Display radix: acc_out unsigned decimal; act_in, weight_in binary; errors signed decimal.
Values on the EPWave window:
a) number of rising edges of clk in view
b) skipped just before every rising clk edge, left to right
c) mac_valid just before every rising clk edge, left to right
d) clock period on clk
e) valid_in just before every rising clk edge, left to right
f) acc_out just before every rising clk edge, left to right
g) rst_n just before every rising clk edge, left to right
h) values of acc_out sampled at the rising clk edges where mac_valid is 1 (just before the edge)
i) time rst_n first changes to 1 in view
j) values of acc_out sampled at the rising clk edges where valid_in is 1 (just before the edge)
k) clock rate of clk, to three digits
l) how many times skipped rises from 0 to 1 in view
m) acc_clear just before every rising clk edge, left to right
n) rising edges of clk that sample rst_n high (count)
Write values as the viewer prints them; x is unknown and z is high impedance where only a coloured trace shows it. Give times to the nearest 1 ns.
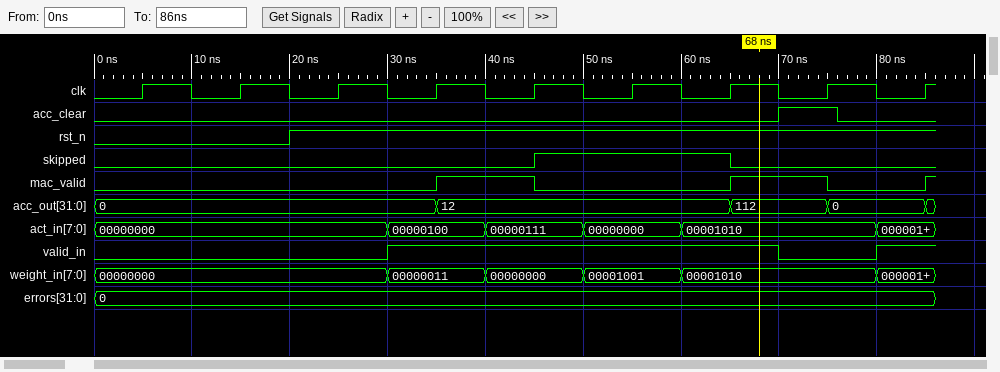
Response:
9
0 0 0 0 0 1 1 0 0
0 0 0 0 1 0 0 1 0
10 ns
0 0 0 1 1 1 1 0 1
0, 0, 0, 0, 12, 12, 12, 112, 0
0 0 1 1 1 1 1 1 1
12, 112
20 ns
0, 12, 12, 12, 0
100 MHz
1
0 0 0 0 0 0 0 1 0
7
